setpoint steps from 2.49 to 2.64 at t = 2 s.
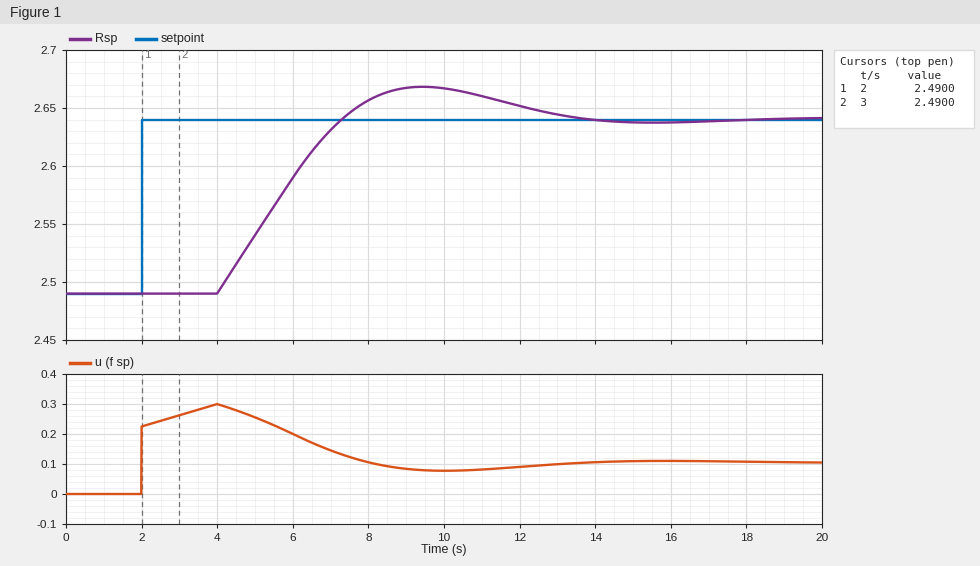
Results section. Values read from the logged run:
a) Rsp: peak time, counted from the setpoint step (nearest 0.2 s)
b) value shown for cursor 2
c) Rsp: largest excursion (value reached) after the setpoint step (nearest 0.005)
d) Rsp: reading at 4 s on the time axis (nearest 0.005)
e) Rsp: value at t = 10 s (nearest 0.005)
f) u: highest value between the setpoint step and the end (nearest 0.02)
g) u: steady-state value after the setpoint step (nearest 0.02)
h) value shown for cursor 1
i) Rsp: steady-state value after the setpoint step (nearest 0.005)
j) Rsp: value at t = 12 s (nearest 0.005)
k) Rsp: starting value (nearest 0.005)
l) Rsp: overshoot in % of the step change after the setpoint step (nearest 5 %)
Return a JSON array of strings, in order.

["7.4 s", "2.4900", "2.670", "2.490", "2.665", "0.30", "0.10", "2.4900", "2.640", "2.650", "2.490", "20 %"]
